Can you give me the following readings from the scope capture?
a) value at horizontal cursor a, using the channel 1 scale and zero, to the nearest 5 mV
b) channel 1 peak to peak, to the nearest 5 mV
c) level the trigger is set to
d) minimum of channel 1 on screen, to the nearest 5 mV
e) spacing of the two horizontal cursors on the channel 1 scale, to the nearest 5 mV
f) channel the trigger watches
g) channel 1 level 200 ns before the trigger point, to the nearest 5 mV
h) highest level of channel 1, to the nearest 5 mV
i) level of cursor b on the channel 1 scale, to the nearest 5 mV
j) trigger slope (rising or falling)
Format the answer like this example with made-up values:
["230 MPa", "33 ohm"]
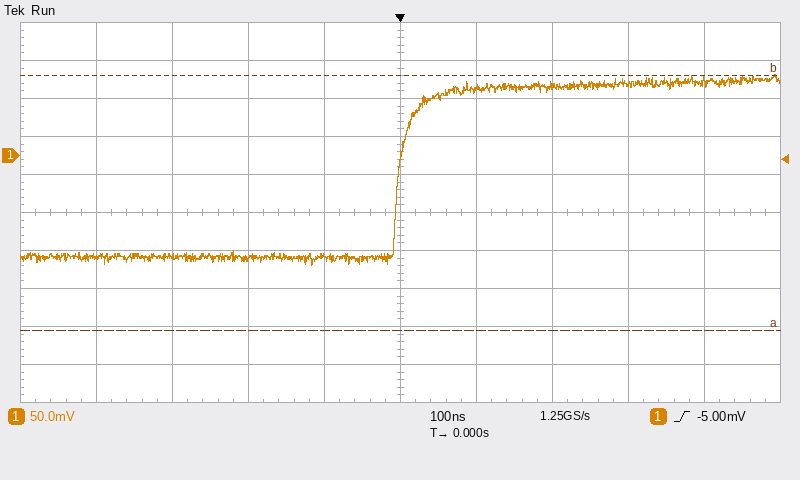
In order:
["-230 mV", "250 mV", "-5.00 mV", "-145 mV", "335 mV", "channel 1", "-135 mV", "105 mV", "105 mV", "rising"]
